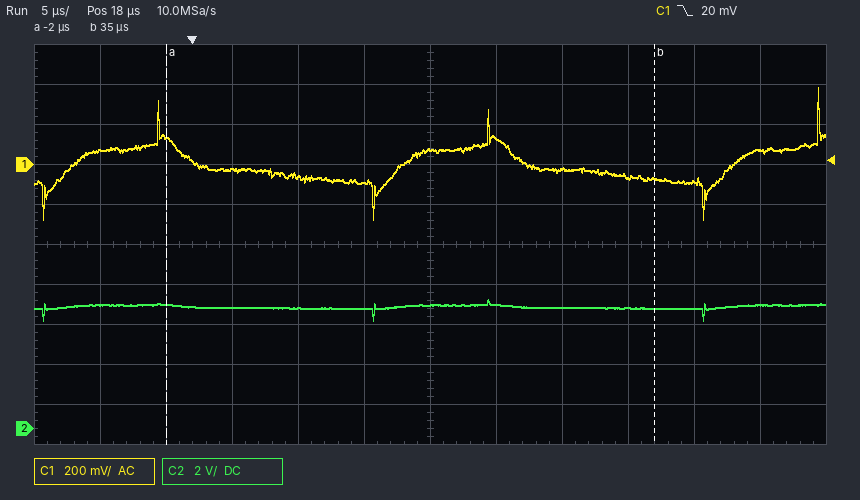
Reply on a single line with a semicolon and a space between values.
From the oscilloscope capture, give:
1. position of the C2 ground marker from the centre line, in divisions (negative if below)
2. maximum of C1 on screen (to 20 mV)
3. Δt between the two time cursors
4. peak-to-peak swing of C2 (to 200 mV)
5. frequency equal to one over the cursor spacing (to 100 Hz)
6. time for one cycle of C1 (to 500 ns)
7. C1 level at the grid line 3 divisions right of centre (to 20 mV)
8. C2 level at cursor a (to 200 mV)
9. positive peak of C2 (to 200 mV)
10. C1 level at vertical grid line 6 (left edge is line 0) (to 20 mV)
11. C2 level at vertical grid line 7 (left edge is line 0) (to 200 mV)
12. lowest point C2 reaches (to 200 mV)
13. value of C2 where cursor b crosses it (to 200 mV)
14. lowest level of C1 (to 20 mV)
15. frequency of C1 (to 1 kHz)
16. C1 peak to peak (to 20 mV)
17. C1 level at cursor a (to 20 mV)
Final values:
-4.6 div; 380 mV; 37.0 µs; 1.0 V; 27.0 kHz; 25.0 µs; -60 mV; 6.2 V; 6.4 V; 80 mV; 6.2 V; 5.4 V; 6.0 V; -280 mV; 40 kHz; 660 mV; 140 mV
